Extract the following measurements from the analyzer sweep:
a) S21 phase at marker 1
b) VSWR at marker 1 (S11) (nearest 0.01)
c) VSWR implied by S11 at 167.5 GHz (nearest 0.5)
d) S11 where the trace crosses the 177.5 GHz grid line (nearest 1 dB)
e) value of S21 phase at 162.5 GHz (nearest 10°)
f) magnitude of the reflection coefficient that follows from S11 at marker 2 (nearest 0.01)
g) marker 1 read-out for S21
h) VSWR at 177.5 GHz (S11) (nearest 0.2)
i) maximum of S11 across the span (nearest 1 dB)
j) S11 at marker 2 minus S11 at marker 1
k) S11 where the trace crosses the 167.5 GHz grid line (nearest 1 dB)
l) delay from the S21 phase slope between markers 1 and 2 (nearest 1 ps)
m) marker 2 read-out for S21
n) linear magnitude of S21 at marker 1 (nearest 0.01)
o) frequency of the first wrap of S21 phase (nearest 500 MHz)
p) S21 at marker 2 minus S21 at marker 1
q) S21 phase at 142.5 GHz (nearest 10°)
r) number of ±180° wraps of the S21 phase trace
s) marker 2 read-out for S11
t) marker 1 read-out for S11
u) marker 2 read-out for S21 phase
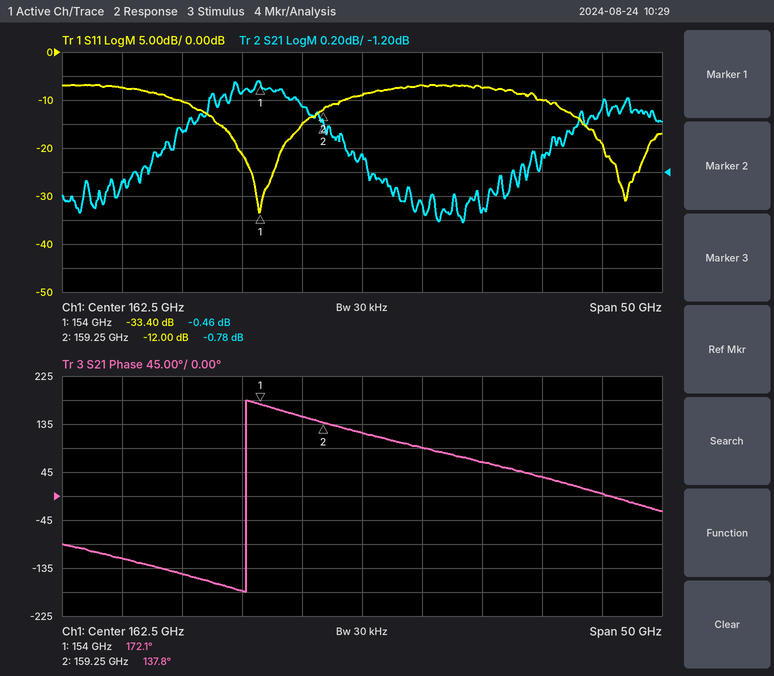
172.1°
1.04
2.5
-10 dB
120°
0.25
-0.46 dB
2.0
-7 dB
21.40 dB
-7 dB
18 ps
-0.78 dB
0.95
153.0 GHz
-0.32 dB
-120°
1
-12.00 dB
-33.40 dB
137.8°
